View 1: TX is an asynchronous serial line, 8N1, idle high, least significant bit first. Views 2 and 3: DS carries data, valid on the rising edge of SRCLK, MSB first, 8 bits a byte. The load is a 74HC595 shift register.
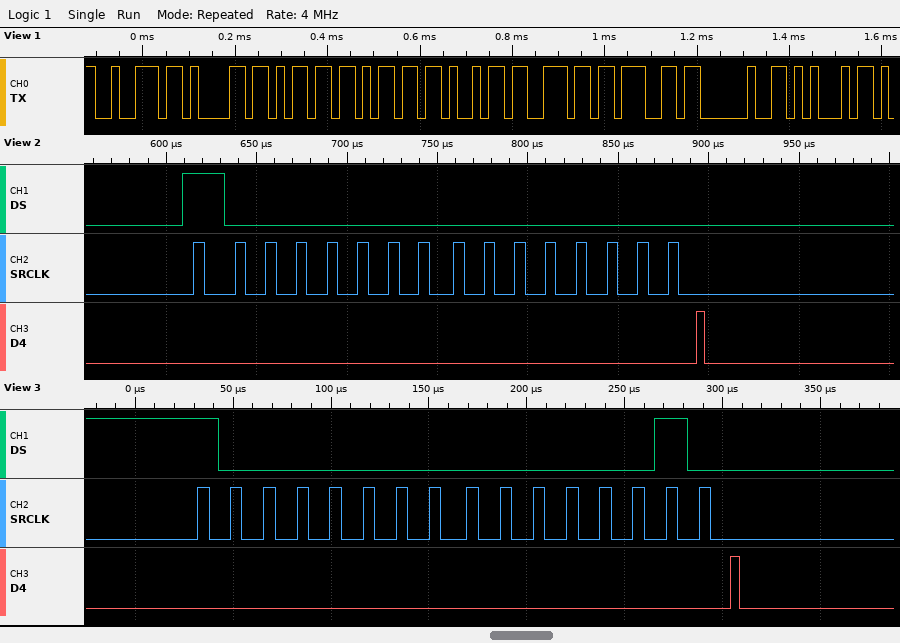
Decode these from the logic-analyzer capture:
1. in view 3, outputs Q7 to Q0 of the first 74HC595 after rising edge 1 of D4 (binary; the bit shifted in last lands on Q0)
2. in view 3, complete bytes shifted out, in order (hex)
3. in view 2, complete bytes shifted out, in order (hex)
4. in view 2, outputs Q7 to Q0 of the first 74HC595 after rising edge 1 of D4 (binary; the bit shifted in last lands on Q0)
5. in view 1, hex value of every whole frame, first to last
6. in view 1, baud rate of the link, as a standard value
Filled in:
00000010
80 02
0x80 0x00
00000000
0x72 0x61 0x6D 0x6D 0x69 0x6E 0x67 0x20 0x45
57600 baud
